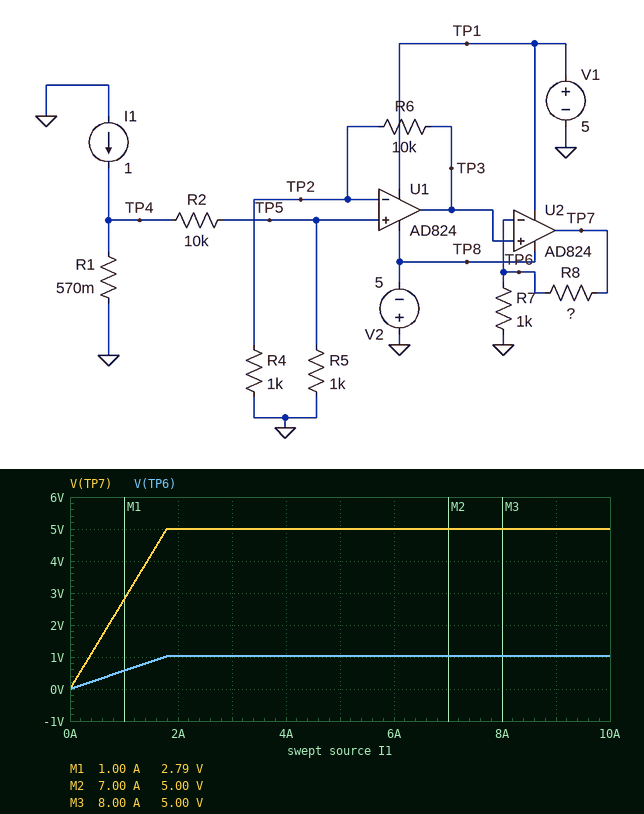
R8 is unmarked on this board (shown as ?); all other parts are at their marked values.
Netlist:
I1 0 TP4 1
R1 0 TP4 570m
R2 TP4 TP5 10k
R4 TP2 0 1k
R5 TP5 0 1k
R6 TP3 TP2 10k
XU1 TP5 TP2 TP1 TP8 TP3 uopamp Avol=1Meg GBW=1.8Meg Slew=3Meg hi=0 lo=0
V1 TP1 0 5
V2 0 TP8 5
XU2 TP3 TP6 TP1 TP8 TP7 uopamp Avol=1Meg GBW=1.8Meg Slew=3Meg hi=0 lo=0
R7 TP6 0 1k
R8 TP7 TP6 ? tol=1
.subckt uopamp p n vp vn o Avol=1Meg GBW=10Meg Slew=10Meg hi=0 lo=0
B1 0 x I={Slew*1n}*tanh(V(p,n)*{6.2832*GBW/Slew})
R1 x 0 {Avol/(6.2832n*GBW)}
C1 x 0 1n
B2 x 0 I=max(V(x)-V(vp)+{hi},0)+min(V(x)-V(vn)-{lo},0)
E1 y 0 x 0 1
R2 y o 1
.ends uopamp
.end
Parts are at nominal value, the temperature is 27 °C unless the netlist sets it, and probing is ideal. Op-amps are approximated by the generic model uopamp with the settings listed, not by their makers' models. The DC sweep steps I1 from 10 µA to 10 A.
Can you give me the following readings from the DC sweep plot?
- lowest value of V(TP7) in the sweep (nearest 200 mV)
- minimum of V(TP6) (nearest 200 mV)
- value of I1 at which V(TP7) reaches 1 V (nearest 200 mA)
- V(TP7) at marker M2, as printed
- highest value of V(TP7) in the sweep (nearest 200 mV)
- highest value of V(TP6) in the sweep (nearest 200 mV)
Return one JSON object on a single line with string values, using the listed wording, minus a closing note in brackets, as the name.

{"lowest value of V(TP7) in the sweep": "0 V", "minimum of V(TP6)": "0 V", "value of I1 at which V(TP7) reaches 1 V": "400 mA", "V(TP7) at marker M2, as printed": "5.00 V", "highest value of V(TP7) in the sweep": "5.0 V", "highest value of V(TP6) in the sweep": "1.0 V"}
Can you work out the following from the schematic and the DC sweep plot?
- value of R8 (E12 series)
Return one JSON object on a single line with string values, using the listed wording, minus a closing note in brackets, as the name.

{"value of R8": "3.9 kΩ"}
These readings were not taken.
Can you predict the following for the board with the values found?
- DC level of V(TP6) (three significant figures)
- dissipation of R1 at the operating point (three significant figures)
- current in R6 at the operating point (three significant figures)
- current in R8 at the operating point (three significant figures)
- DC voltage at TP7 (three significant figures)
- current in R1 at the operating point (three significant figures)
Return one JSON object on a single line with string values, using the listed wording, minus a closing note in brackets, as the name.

{"DC level of V(TP6)": "570 mV", "dissipation of R1 at the operating point": "570 mW", "current in R6 at the operating point": "51.8 µA", "current in R8 at the operating point": "570 µA", "DC voltage at TP7": "2.79 V", "current in R1 at the operating point": "1.00 A"}
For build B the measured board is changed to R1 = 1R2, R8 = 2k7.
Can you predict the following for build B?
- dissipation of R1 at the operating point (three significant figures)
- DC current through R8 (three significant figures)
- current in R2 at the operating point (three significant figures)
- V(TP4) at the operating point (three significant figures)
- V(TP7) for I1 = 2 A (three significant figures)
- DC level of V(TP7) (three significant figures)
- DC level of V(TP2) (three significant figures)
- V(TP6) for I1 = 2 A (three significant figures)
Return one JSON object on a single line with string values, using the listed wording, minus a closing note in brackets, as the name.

{"dissipation of R1 at the operating point": "1.20 W", "DC current through R8": "1.20 mA", "current in R2 at the operating point": "109 µA", "V(TP4) at the operating point": "1.20 V", "V(TP7) for I1 = 2 A": "5.00 V", "DC level of V(TP7)": "4.44 V", "DC level of V(TP2)": "109 mV", "V(TP6) for I1 = 2 A": "1.35 V"}
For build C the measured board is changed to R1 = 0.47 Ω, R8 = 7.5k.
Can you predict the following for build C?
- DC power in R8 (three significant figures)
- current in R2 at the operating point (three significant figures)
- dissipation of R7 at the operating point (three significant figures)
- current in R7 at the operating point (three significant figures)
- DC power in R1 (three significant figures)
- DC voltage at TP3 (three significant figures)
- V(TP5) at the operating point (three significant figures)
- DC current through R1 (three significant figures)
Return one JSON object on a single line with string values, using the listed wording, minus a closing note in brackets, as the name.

{"DC power in R8": "1.66 mW", "current in R2 at the operating point": "42.7 µA", "dissipation of R7 at the operating point": "221 µW", "current in R7 at the operating point": "470 µA", "DC power in R1": "470 mW", "DC voltage at TP3": "470 mV", "V(TP5) at the operating point": "42.7 mV", "DC current through R1": "1.00 A"}
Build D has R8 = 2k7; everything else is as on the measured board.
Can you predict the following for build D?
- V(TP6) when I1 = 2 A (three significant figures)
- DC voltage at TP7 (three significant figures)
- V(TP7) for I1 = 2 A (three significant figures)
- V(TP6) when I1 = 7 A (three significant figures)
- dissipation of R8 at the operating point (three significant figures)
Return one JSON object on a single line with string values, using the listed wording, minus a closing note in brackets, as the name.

{"V(TP6) when I1 = 2 A": "1.14 V", "DC voltage at TP7": "2.11 V", "V(TP7) for I1 = 2 A": "4.22 V", "V(TP6) when I1 = 7 A": "1.35 V", "dissipation of R8 at the operating point": "877 µW"}
